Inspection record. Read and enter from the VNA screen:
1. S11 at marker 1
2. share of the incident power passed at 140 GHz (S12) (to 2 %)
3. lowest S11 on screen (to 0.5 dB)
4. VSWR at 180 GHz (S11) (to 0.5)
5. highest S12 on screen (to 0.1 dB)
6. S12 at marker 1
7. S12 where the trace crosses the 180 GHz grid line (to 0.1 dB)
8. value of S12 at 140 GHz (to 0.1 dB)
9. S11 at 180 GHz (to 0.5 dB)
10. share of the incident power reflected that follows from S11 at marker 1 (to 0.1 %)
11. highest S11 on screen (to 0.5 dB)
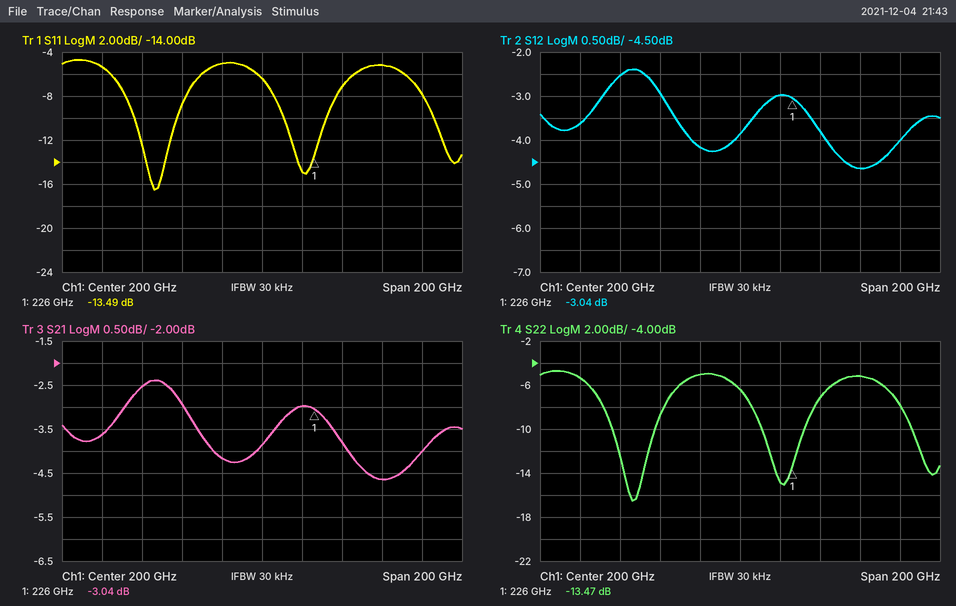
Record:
-13.49 dB
56 %
-16.5 dB
3.5
-2.4 dB
-3.04 dB
-4.2 dB
-2.5 dB
-5.0 dB
4.5 %
-4.5 dB
